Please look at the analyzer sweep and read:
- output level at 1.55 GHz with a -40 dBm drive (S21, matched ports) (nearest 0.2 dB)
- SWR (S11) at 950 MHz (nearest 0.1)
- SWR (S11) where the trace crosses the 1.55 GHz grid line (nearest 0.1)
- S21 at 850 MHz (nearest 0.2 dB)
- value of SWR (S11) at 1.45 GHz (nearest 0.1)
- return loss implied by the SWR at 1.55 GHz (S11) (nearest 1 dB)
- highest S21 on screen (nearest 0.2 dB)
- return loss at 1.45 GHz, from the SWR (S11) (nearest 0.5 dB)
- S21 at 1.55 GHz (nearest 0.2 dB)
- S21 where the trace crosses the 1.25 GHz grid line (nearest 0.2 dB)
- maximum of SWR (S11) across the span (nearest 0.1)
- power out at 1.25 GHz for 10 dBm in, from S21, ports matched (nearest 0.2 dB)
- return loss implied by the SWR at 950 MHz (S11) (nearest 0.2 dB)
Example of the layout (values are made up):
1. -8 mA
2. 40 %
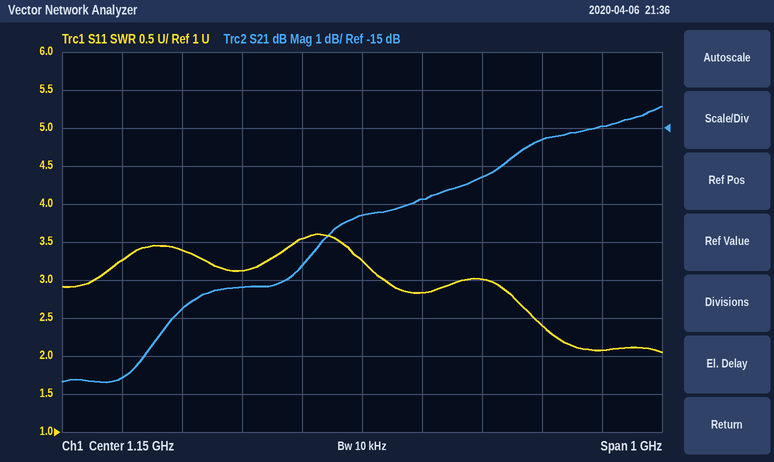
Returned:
1. -55.0 dBm
2. 3.1
3. 2.1
4. -19.8 dB
5. 2.4
6. 9 dB
7. -14.4 dB
8. 7.5 dB
9. -15.0 dB
10. -16.8 dB
11. 3.6
12. -6.8 dBm
13. 5.8 dB
